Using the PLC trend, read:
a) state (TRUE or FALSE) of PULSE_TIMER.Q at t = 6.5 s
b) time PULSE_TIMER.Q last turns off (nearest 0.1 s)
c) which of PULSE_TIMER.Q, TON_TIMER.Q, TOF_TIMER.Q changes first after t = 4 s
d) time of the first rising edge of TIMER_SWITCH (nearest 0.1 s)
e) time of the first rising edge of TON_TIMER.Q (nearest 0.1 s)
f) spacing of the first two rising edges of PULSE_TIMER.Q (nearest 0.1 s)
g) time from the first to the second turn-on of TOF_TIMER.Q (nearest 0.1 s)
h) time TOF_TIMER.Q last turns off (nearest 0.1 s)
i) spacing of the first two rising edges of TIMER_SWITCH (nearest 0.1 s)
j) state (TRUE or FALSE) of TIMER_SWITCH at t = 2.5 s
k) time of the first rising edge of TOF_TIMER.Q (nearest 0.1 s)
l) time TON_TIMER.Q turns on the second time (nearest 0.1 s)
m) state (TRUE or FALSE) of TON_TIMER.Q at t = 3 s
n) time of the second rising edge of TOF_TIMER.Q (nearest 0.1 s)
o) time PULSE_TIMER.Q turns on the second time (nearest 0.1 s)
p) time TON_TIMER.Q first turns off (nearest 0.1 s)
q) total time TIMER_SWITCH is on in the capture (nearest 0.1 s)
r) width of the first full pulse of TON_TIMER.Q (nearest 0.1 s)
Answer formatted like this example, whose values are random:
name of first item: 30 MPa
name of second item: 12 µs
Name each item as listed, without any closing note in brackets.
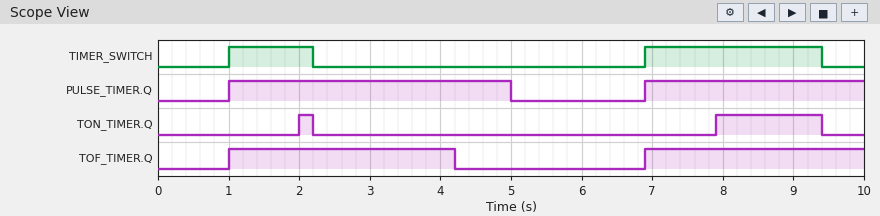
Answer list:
state (TRUE or FALSE) of PULSE_TIMER.Q at t = 6.5 s: FALSE
time PULSE_TIMER.Q last turns off: 5.0 s
which of PULSE_TIMER.Q, TON_TIMER.Q, TOF_TIMER.Q changes first after t = 4 s: TOF_TIMER.Q
time of the first rising edge of TIMER_SWITCH: 1.0 s
time of the first rising edge of TON_TIMER.Q: 2.0 s
spacing of the first two rising edges of PULSE_TIMER.Q: 5.9 s
time from the first to the second turn-on of TOF_TIMER.Q: 5.9 s
time TOF_TIMER.Q last turns off: 4.2 s
spacing of the first two rising edges of TIMER_SWITCH: 5.9 s
state (TRUE or FALSE) of TIMER_SWITCH at t = 2.5 s: FALSE
time of the first rising edge of TOF_TIMER.Q: 1.0 s
time TON_TIMER.Q turns on the second time: 7.9 s
state (TRUE or FALSE) of TON_TIMER.Q at t = 3 s: FALSE
time of the second rising edge of TOF_TIMER.Q: 6.9 s
time PULSE_TIMER.Q turns on the second time: 6.9 s
time TON_TIMER.Q first turns off: 2.2 s
total time TIMER_SWITCH is on in the capture: 3.7 s
width of the first full pulse of TON_TIMER.Q: 0.2 s
